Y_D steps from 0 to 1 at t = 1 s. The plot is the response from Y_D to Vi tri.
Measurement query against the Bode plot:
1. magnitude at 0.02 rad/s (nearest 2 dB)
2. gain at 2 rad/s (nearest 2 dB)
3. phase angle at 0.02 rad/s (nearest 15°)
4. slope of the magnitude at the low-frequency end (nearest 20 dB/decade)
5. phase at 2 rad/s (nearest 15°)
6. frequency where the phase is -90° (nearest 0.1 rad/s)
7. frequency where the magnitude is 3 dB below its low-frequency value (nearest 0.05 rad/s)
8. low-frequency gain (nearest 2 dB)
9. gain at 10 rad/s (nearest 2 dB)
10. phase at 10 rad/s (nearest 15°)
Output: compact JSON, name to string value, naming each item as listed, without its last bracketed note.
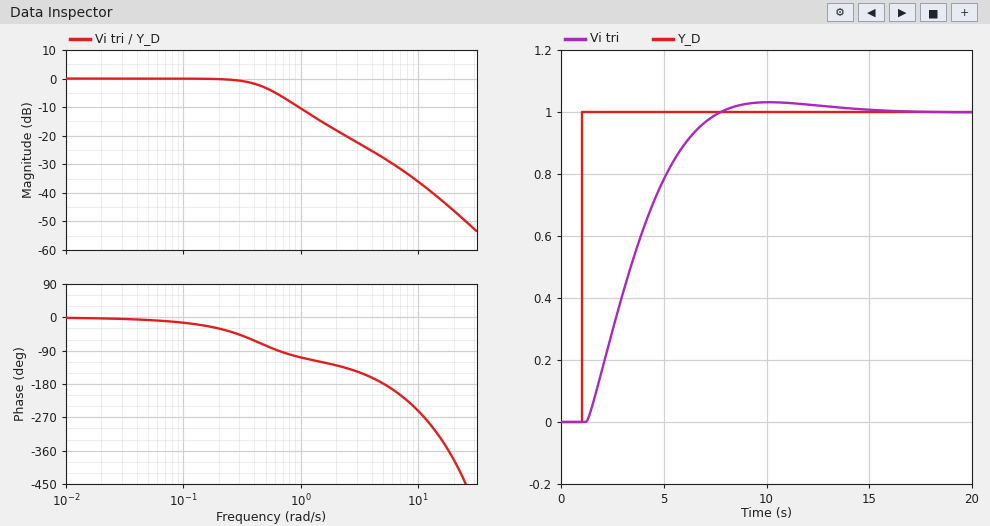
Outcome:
{"magnitude at 0.02 rad/s": "0 dB", "gain at 2 rad/s": "-18 dB", "phase angle at 0.02 rad/s": "0°", "slope of the magnitude at the low-frequency end": "0 dB/decade", "phase at 2 rad/s": "-135°", "frequency where the phase is -90°": "0.6 rad/s", "frequency where the magnitude is 3 dB below its low-frequency value": "0.50 rad/s", "low-frequency gain": "0 dB", "gain at 10 rad/s": "-36 dB", "phase at 10 rad/s": "-255°"}
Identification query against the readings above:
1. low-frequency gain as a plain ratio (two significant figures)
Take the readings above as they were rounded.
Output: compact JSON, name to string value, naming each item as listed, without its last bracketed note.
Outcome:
{"low-frequency gain as a plain ratio": "1.0"}
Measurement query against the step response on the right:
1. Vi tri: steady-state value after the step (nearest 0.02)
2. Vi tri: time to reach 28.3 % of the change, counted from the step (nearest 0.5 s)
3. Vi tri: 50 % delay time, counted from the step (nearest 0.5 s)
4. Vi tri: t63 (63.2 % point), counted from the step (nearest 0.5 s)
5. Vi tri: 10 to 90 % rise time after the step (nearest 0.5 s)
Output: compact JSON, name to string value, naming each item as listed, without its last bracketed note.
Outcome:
{"Vi tri: steady-state value after the step": "1.00", "Vi tri: time to reach 28.3 % of the change, counted from the step": "1.5 s", "Vi tri: 50 % delay time, counted from the step": "2.5 s", "Vi tri: t63 (63.2 % point), counted from the step": "3.0 s", "Vi tri: 10 to 90 % rise time after the step": "4.5 s"}
